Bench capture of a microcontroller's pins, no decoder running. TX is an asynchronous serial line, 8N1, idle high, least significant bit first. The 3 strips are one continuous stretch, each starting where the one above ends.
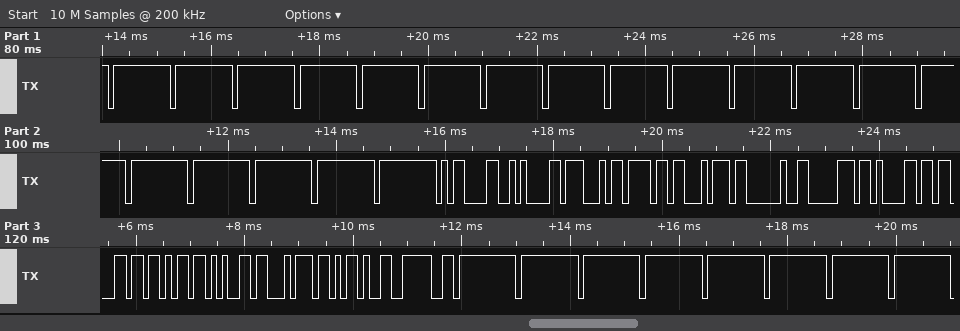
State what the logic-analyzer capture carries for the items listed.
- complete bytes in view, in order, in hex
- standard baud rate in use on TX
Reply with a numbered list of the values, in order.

1. FF FF FF FF FF FF FF FF FF FF FF FF FF FF FF FF FF FF FF 0D 0A 47 6F 74 20 70 61 63 6B 65 74 2D 3E FF FF FF FF FF FF FF FF
2. 9600 baud
